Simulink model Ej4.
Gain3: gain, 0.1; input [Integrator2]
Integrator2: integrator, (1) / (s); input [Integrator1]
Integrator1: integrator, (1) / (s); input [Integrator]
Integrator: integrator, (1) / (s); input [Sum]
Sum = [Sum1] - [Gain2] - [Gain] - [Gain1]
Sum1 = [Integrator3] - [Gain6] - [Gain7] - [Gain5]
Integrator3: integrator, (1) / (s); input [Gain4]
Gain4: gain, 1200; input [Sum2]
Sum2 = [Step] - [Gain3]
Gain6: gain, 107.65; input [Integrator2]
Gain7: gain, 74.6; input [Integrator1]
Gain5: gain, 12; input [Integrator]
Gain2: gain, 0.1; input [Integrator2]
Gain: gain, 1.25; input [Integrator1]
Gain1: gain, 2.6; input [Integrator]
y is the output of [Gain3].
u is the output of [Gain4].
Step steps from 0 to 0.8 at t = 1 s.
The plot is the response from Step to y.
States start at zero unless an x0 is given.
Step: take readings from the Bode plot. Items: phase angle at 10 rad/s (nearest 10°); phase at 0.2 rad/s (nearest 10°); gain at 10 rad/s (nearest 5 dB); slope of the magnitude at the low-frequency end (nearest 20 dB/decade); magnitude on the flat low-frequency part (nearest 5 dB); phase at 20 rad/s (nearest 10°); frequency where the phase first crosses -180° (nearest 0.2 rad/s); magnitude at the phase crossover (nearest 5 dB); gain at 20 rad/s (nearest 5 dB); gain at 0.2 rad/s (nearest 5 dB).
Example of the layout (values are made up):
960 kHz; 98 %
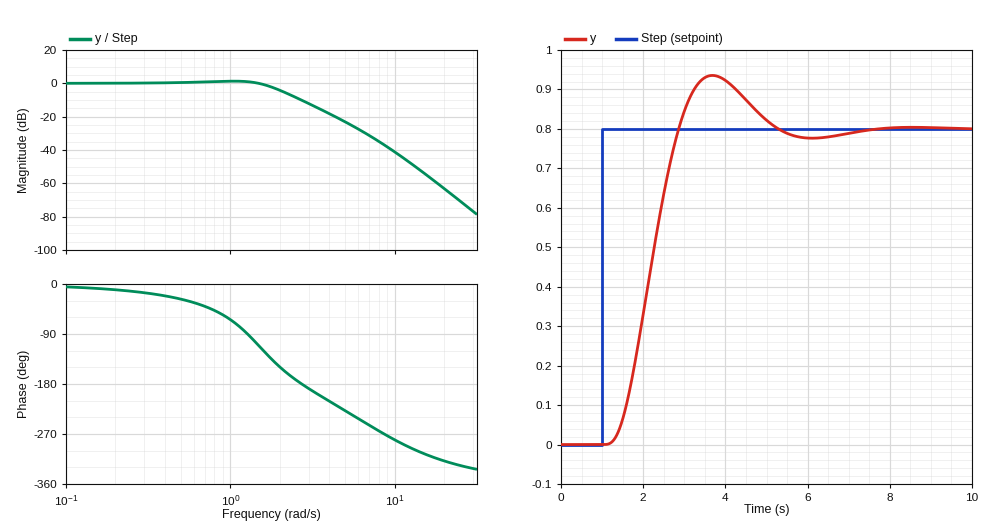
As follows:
-280°; -10°; -40 dB; 0 dB/decade; 0 dB; -320°; 2.8 rad/s; -10 dB; -65 dB; 0 dB
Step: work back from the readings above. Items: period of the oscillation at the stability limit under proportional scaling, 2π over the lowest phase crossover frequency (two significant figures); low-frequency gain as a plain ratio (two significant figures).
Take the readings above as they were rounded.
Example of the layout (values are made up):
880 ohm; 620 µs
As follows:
2.2 s; 1.0
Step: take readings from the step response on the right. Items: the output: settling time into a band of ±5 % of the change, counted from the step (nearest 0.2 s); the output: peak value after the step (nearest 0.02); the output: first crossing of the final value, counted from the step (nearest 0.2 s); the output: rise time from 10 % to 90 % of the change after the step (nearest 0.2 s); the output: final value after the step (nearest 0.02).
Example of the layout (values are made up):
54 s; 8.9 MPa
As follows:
3.8 s; 0.94; 1.8 s; 1.2 s; 0.80
